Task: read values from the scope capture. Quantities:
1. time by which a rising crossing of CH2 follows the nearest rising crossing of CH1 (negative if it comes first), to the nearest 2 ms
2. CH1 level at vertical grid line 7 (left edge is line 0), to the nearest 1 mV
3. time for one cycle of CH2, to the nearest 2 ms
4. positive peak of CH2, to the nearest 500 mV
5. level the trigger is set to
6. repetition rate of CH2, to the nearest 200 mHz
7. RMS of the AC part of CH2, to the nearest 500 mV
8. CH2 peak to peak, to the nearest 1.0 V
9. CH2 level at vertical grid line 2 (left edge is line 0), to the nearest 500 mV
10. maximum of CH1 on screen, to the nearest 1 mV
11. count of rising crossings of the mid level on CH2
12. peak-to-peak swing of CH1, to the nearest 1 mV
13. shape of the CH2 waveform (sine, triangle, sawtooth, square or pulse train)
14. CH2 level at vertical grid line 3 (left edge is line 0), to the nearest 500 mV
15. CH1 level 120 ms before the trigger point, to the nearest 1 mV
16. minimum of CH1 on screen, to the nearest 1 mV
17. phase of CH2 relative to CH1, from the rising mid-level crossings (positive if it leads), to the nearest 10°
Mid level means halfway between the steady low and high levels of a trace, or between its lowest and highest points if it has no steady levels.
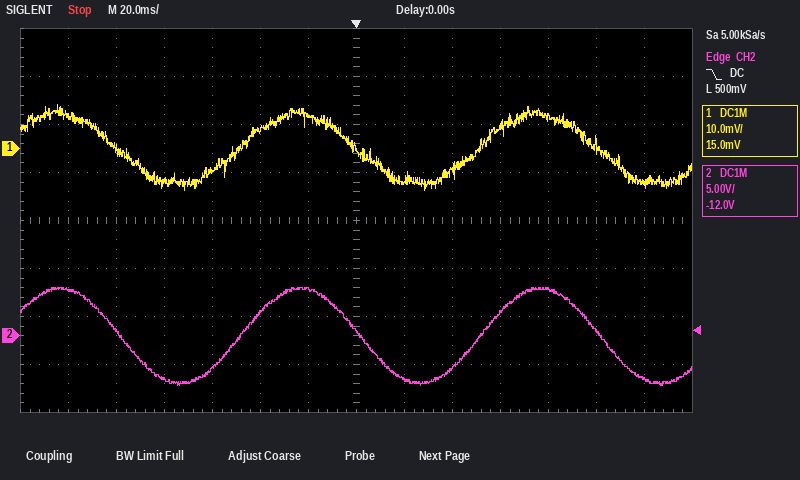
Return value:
0 ms
0 mV
100 ms
5.0 V
500 mV
10.0 Hz
3.5 V
10.0 V
500 mV
9 mV
2
18 mV
sine
-4.5 V
7 mV
-9 mV
0°
